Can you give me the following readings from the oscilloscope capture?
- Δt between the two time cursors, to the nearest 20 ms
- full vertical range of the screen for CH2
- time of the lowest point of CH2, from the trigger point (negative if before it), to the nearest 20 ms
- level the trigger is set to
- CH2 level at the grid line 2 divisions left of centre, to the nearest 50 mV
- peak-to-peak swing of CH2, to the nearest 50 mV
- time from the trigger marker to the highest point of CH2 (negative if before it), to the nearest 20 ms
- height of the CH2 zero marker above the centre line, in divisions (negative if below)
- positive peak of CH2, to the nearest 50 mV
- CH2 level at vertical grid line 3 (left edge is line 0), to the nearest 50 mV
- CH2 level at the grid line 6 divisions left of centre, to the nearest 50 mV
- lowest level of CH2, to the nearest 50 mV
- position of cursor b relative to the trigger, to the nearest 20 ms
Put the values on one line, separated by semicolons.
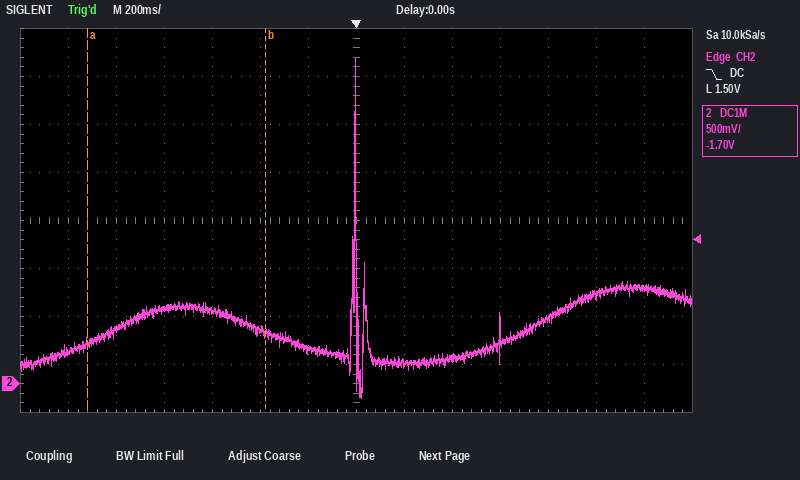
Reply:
740 ms; 4 V; +20 ms; 1.50 V; 550 mV; 3.55 V; 0 ms; -3.4 div; 3.40 V; 800 mV; 350 mV; -150 mV; -380 ms
